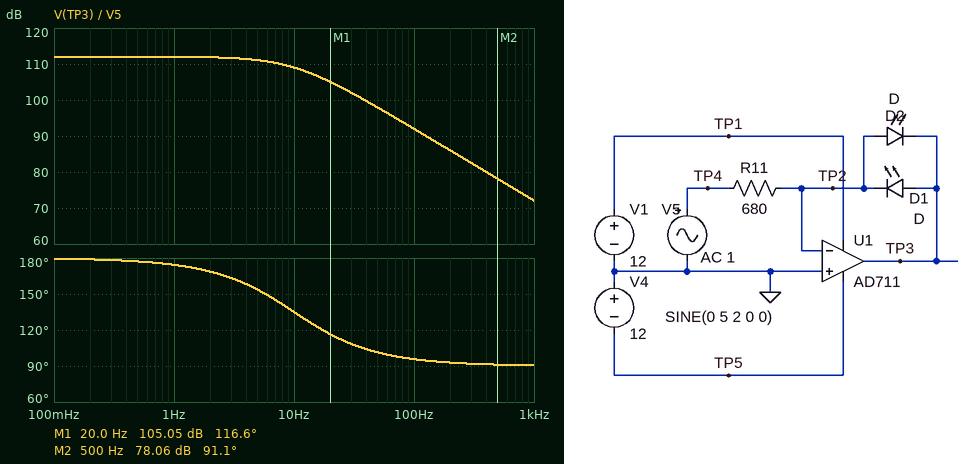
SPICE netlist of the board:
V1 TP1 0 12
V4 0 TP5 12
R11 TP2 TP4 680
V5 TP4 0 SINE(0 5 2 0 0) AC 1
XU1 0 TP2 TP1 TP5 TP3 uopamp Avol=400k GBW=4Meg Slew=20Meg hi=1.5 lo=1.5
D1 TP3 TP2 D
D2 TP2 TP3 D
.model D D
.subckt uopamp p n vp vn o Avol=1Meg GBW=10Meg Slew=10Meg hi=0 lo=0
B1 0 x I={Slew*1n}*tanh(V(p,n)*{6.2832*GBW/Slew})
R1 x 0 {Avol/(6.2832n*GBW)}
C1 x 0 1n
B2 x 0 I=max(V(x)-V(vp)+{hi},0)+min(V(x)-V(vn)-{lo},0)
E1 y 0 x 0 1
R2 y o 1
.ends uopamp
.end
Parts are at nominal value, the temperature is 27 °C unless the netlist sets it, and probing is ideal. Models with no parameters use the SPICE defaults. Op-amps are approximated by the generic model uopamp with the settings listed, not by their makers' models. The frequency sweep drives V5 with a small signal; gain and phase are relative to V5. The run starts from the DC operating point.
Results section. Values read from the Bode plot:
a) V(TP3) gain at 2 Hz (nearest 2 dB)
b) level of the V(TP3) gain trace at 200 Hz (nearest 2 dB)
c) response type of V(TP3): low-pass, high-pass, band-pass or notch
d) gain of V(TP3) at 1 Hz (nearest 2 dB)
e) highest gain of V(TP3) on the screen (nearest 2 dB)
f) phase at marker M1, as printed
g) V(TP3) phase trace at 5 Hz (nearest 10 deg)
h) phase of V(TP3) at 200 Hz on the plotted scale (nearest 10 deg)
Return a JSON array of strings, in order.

["112 dB", "86 dB", "low-pass", "112 dB", "112 dB", "116.6 deg", "150 deg", "90 deg"]
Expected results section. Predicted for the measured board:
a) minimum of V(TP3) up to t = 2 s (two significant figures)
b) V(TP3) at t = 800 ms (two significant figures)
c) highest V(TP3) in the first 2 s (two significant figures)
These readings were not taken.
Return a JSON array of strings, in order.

["-710 mV", "690 mV", "710 mV"]
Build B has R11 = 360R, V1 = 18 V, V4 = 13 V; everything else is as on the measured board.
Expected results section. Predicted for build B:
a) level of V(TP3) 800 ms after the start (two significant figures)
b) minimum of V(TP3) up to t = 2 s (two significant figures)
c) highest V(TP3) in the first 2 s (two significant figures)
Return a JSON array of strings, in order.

["710 mV", "-720 mV", "720 mV"]
